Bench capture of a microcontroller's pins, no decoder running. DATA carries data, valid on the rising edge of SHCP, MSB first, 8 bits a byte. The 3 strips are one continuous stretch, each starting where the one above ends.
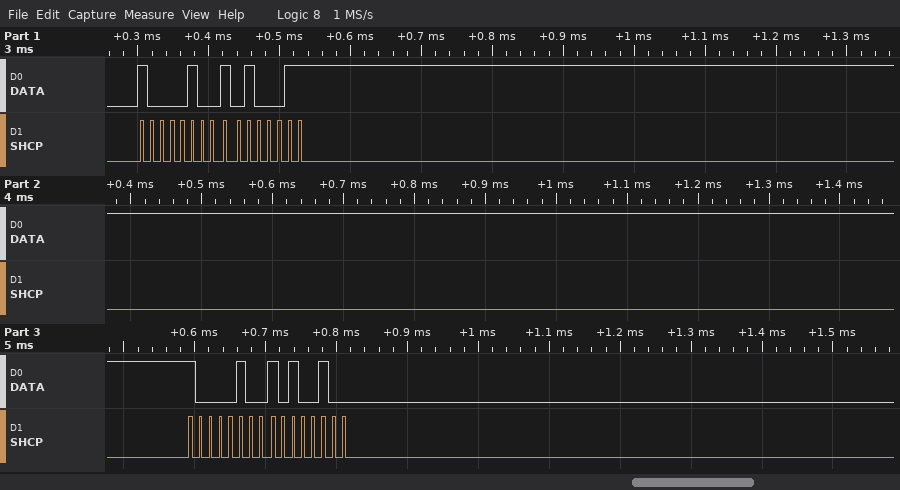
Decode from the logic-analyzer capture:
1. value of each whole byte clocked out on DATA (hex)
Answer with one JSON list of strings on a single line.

["84 A3 84 A4"]
